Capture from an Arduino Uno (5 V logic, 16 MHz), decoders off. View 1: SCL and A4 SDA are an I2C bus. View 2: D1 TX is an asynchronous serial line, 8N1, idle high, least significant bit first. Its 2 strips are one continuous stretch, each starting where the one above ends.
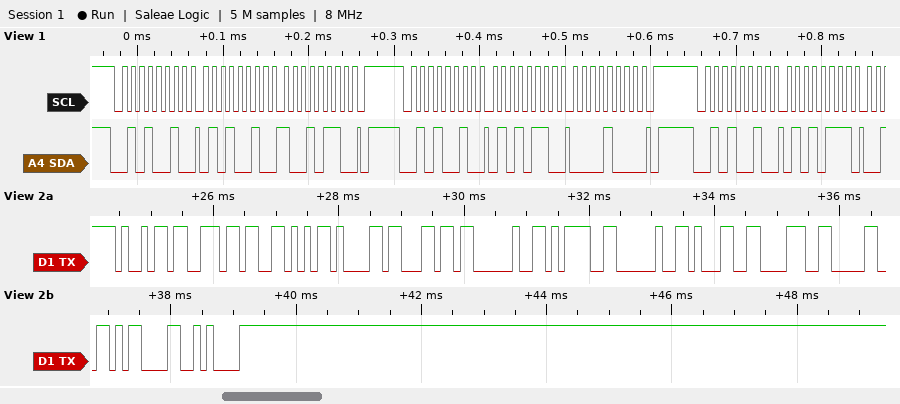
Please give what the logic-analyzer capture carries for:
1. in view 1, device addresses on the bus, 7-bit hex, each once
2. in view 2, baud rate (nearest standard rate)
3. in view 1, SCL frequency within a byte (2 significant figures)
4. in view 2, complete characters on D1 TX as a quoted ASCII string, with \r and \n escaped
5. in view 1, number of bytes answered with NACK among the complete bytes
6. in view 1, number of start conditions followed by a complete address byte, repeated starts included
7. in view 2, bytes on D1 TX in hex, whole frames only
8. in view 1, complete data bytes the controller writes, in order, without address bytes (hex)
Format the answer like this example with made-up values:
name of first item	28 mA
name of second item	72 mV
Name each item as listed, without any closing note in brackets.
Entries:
in view 1, device addresses on the bus, 7-bit hex, each once	0x29
in view 2, baud rate	9600 baud
in view 1, SCL frequency within a byte	100 kHz
in view 2, complete characters on D1 TX as a quoted ASCII string, with \r and \n escaped	"inVal = 180\r\n"
in view 1, number of bytes answered with NACK among the complete bytes	0
in view 1, number of start conditions followed by a complete address byte, repeated starts included	3
in view 2, bytes on D1 TX in hex, whole frames only	69 6E 56 61 6C 20 3D 20 31 38 30 0D 0A
in view 1, complete data bytes the controller writes, in order, without address bytes	52 96 56 08 57
